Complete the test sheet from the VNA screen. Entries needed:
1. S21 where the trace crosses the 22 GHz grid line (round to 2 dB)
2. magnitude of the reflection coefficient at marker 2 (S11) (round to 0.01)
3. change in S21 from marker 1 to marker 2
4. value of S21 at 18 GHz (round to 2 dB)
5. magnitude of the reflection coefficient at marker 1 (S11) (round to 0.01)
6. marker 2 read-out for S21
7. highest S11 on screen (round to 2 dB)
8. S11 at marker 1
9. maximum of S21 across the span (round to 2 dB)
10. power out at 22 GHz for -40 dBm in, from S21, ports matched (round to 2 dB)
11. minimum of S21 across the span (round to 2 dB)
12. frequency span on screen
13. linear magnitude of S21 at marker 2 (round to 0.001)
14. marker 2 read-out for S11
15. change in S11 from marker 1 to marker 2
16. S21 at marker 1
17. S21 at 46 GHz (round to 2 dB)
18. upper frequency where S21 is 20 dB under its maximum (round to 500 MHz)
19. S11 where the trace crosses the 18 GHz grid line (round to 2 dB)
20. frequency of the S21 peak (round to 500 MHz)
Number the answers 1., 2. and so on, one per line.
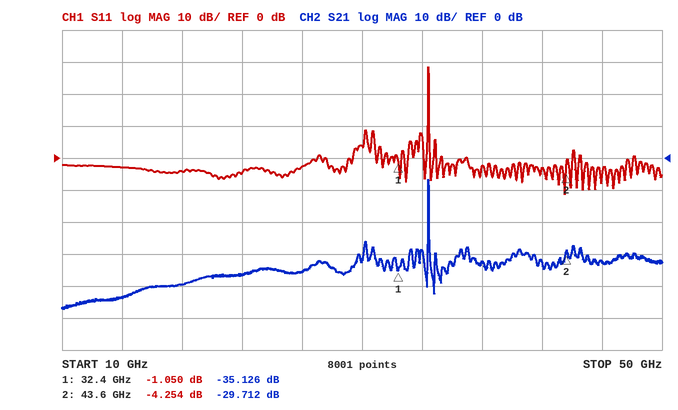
1. -36 dB
2. 0.61
3. 5.414 dB
4. -40 dB
5. 0.89
6. -29.712 dB
7. 28 dB
8. -1.050 dB
9. -6 dB
10. -76 dBm
11. -48 dB
12. 40 GHz
13. 0.033
14. -4.254 dB
15. -3.204 dB
16. -35.126 dB
17. -32 dB
18. 34.5 GHz
19. -4 dB
20. 34.5 GHz
